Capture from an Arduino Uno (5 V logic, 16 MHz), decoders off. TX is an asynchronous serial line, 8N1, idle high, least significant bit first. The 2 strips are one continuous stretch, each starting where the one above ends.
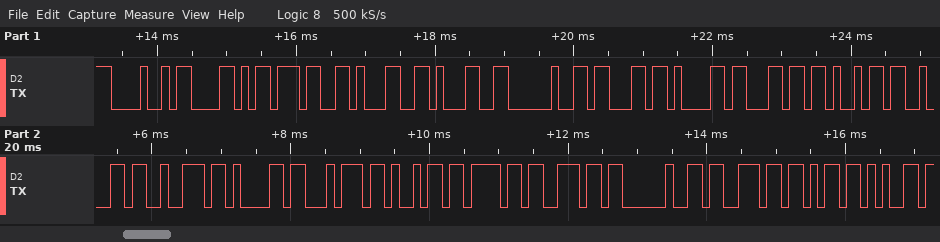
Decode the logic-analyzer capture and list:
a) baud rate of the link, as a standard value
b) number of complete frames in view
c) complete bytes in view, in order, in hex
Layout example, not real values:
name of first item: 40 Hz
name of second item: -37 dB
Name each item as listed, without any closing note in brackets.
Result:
baud rate of the link, as a standard value: 9600 baud
number of complete frames in view: 21
complete bytes in view, in order, in hex: 0x48 0x58 0x37 0x31 0x31 0x20 0x63 0x61 0x6C 0x69 0x62 0x72 0x61 0x74 0x69 0x6F 0x6E 0x20 0x73 0x6B 0x65
